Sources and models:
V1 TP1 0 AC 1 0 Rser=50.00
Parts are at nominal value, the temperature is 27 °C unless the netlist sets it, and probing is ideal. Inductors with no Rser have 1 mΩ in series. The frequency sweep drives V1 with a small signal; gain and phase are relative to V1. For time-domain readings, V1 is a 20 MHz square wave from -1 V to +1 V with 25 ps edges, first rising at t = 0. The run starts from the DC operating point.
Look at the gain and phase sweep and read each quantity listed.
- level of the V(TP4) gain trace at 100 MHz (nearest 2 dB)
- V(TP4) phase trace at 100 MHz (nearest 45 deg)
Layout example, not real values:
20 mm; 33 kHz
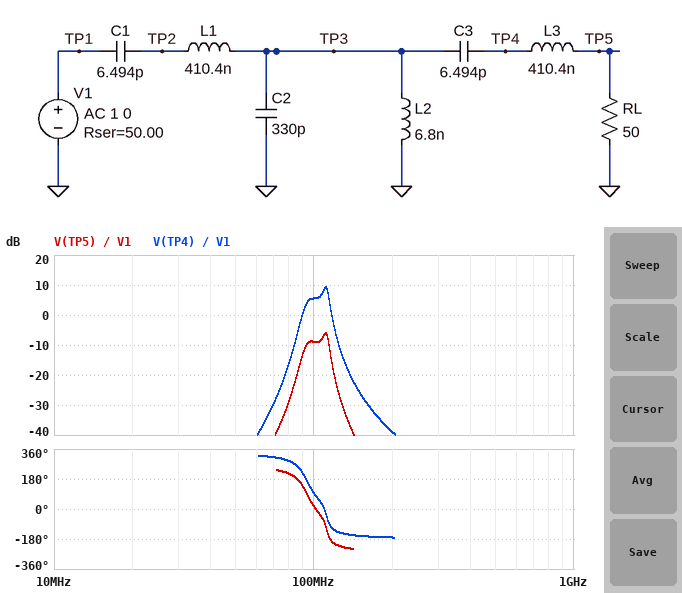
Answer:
6 dB; 90 deg
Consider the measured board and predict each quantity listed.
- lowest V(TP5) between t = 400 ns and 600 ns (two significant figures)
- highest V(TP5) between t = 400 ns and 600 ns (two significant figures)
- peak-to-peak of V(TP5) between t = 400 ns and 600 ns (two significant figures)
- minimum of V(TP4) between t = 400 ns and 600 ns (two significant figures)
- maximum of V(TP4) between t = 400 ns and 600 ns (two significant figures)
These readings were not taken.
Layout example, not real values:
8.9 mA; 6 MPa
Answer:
-95 mV; 95 mV; 190 mV; -500 mV; 500 mV
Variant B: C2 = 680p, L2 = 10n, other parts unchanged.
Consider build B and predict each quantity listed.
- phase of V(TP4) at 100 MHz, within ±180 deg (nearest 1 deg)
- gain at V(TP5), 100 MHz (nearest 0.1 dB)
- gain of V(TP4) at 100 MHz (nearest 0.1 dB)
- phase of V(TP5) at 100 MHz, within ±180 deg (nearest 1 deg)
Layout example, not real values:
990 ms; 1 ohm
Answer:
-31 deg; -22.9 dB; -8.5 dB; -110 deg
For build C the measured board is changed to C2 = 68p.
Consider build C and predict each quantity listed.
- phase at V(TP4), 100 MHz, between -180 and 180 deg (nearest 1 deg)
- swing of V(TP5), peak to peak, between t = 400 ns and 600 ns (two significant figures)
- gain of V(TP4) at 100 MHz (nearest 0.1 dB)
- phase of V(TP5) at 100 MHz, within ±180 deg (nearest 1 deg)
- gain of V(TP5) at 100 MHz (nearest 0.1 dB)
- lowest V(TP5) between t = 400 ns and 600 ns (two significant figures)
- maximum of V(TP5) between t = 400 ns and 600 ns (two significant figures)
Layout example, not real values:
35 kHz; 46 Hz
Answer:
130 deg; 54 mV; -6.3 dB; 51 deg; -20.7 dB; -27 mV; 27 mV
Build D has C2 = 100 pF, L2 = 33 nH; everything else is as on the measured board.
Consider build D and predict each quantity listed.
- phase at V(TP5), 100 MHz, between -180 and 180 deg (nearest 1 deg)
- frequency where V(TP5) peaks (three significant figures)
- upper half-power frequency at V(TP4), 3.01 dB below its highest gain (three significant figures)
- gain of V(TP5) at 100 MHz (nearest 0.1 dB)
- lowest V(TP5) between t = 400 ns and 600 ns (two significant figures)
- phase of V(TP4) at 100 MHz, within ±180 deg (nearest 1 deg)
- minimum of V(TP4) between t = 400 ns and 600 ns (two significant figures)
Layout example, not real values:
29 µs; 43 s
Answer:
-36 deg; 104 MHz; 115 MHz; -6.1 dB; -140 mV; 43 deg; -720 mV
